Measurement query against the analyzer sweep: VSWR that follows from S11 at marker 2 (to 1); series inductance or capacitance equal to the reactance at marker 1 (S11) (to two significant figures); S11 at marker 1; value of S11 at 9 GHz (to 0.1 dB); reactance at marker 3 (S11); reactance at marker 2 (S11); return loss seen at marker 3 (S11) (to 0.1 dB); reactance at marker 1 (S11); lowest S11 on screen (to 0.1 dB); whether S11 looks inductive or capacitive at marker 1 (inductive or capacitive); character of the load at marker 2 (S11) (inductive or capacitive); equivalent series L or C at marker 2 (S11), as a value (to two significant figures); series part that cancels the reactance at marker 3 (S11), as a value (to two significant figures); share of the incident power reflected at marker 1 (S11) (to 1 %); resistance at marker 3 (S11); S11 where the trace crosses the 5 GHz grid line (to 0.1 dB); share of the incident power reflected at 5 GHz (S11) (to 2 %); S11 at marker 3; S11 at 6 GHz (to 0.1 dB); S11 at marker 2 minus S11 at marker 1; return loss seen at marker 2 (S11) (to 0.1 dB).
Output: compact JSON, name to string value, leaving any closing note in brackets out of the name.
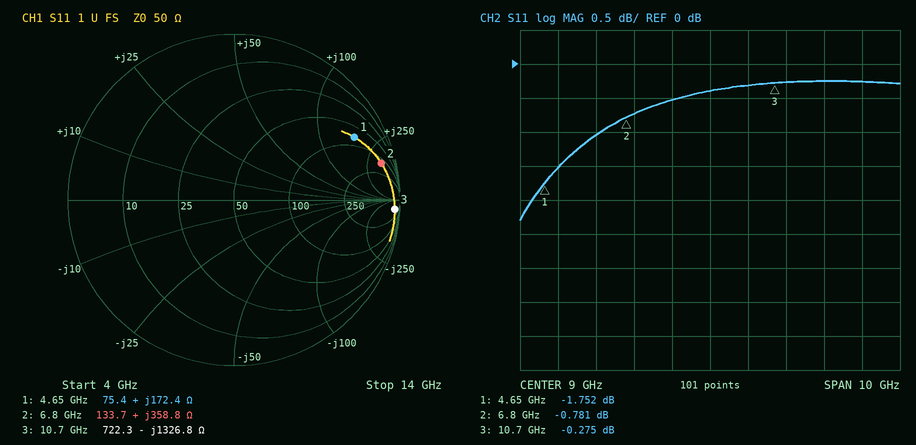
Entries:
{"VSWR that follows from S11 at marker 2": "22", "series inductance or capacitance equal to the reactance at marker 1 (S11)": "5.9 nH", "S11 at marker 1": "-1.752 dB", "value of S11 at 9 GHz": "-0.4 dB", "reactance at marker 3": "-1326.8 Ω", "reactance at marker 2": "+358.8 Ω", "return loss seen at marker 3 (S11)": "0.3 dB", "reactance at marker 1": "+172.4 Ω", "lowest S11 on screen": "-2.3 dB", "whether S11 looks inductive or capacitive at marker 1": "inductive", "character of the load at marker 2 (S11)": "inductive", "equivalent series L or C at marker 2 (S11), as a value": "8.4 nH", "series part that cancels the reactance at marker 3 (S11), as a value": "20 nH", "share of the incident power reflected at marker 1 (S11)": "67 %", "resistance at marker 3": "722.3 Ω", "S11 where the trace crosses the 5 GHz grid line": "-1.5 dB", "share of the incident power reflected at 5 GHz (S11)": "70 %", "S11 at marker 3": "-0.275 dB", "S11 at 6 GHz": "-1.0 dB", "S11 at marker 2 minus S11 at marker 1": "0.971 dB", "return loss seen at marker 2 (S11)": "0.8 dB"}
